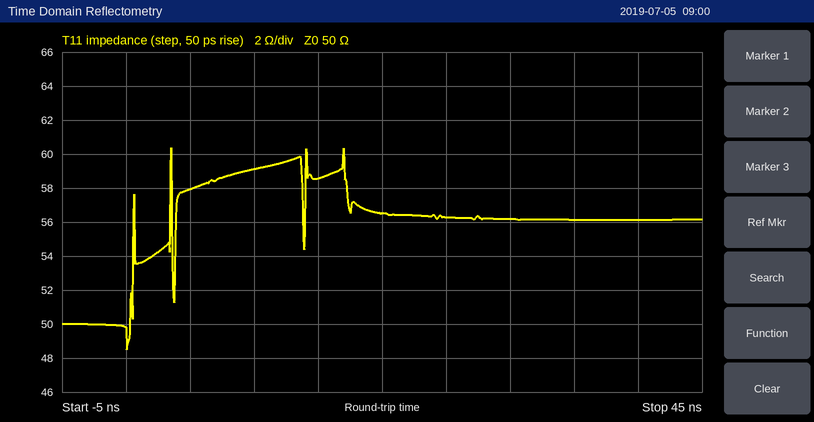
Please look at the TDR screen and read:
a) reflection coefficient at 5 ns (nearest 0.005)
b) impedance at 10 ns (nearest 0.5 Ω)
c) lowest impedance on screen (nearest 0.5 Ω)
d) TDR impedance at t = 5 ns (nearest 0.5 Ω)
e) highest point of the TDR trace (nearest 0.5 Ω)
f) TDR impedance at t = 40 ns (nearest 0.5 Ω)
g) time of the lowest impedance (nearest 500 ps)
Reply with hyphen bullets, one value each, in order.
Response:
- +0.075
- 59.0 Ω
- 48.5 Ω
- 58.0 Ω
- 60.5 Ω
- 56.0 Ω
- 0.0 ns
